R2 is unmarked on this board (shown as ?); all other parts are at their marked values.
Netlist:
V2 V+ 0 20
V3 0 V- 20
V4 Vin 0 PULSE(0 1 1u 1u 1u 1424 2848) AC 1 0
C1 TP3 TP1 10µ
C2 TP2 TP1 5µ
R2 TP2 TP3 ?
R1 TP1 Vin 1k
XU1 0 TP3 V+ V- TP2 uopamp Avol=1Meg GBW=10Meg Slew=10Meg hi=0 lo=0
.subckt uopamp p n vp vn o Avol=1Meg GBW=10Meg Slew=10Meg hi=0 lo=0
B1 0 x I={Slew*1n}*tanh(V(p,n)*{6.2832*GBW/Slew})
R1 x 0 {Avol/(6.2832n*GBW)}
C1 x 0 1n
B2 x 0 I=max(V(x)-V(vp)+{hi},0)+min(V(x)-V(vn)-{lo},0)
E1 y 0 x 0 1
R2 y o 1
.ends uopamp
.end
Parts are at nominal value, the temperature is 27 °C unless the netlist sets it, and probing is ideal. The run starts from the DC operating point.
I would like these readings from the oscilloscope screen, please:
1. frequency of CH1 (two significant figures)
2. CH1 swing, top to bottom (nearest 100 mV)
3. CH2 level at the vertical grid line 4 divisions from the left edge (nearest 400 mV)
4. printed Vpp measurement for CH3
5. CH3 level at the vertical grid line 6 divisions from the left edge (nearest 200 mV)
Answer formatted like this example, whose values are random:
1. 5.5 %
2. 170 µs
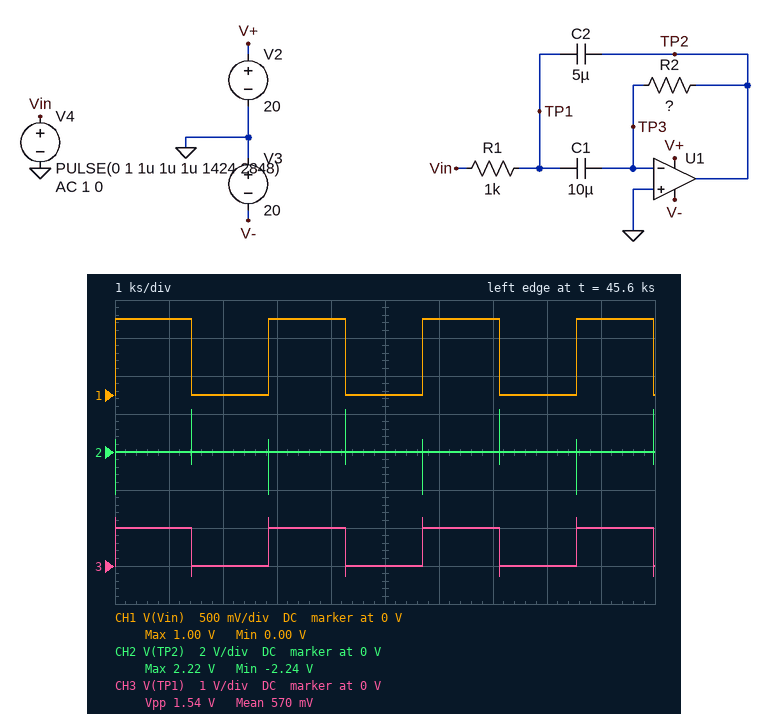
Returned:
1. 350 µHz
2. 1.0 V
3. 0 V
4. 1.54 V
5. 1.0 V
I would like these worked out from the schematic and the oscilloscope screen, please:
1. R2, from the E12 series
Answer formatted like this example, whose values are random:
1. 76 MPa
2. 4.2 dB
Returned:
1. 6.8 kΩ
